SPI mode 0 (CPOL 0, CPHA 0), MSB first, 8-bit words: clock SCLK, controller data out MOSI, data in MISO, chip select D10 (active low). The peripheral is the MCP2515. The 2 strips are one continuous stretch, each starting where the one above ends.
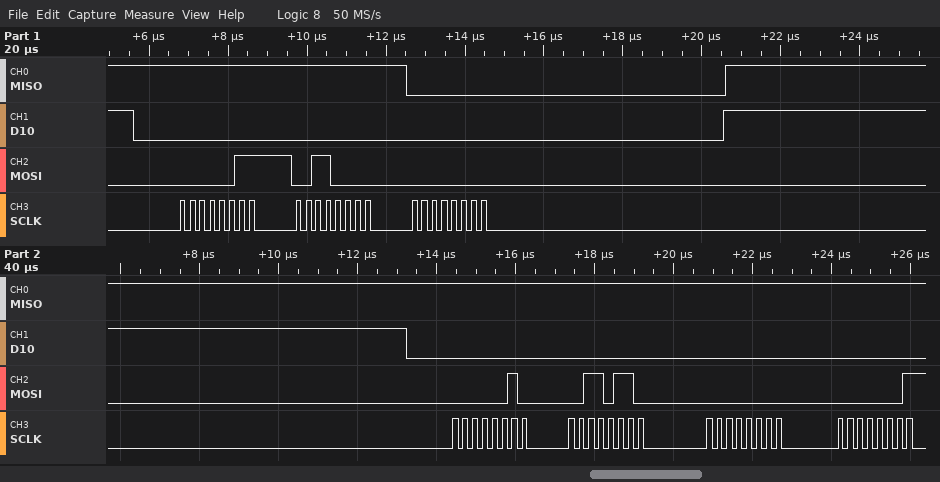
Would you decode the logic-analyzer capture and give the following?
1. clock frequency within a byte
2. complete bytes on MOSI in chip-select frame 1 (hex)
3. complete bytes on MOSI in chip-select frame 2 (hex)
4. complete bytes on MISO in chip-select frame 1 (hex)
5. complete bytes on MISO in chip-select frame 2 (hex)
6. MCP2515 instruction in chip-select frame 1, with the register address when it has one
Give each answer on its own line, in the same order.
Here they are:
4 MHz
03 30 00
02 36 00 01
FF FF 00
FF FF FF FF
READ 0x30
